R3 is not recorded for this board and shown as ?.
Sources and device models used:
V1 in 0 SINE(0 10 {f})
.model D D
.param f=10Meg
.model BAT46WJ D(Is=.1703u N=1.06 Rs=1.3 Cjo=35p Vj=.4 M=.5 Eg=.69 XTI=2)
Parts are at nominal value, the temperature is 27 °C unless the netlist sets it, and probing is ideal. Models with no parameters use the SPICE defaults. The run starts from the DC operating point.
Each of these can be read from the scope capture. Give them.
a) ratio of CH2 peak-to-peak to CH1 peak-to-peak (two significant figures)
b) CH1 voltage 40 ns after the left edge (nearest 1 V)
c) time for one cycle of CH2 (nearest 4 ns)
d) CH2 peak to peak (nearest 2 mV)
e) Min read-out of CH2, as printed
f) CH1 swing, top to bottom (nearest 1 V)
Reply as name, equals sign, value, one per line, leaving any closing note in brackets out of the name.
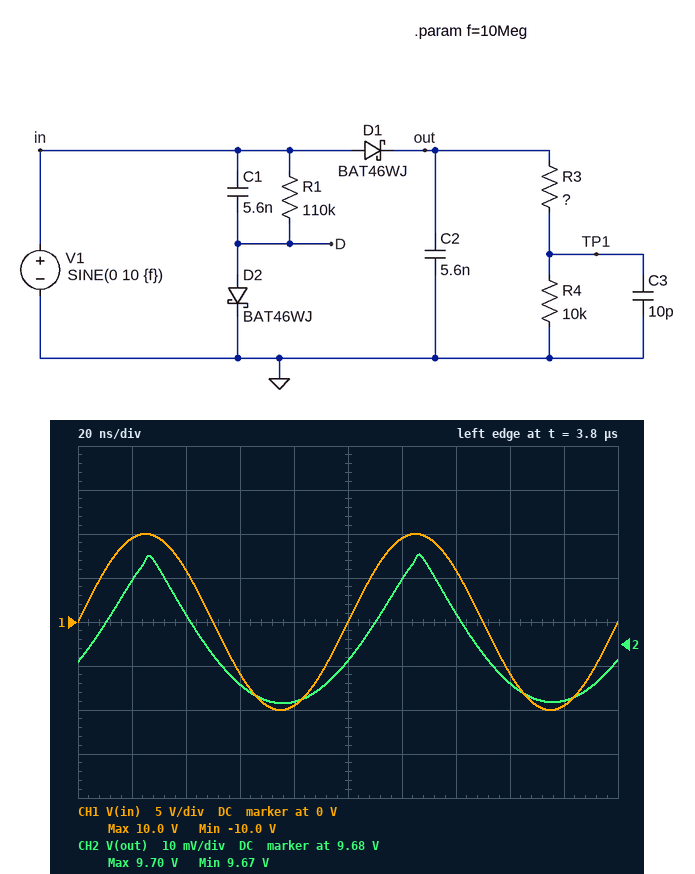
ratio of CH2 peak-to-peak to CH1 peak-to-peak = 0.0017
CH1 voltage 40 ns after the left edge = 6 V
time for one cycle of CH2 = 100 ns
CH2 peak to peak = 34 mV
Min read-out of CH2, as printed = 9.67 V
CH1 swing, top to bottom = 20 V
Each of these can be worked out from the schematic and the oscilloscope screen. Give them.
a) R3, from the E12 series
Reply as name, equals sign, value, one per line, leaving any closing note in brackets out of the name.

R3, from the E12 series = 56 kΩ
